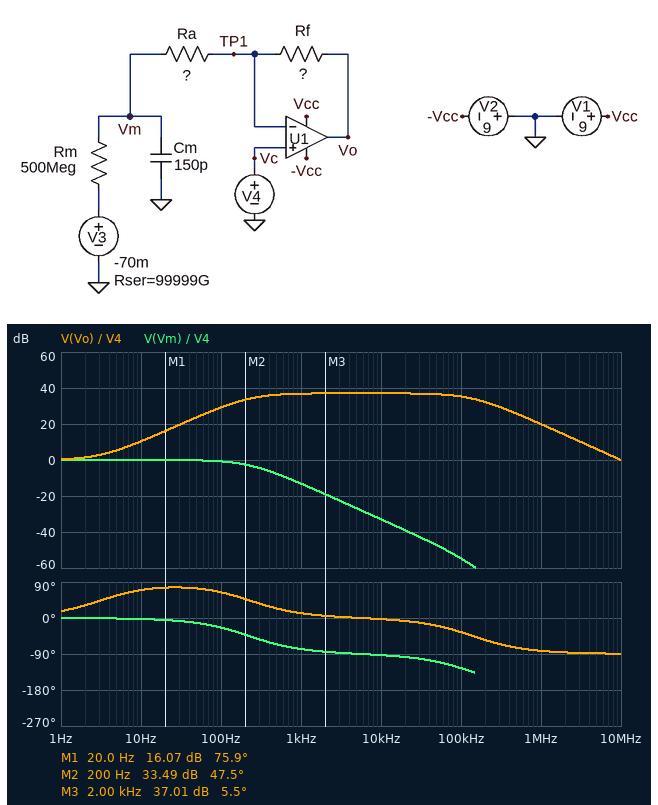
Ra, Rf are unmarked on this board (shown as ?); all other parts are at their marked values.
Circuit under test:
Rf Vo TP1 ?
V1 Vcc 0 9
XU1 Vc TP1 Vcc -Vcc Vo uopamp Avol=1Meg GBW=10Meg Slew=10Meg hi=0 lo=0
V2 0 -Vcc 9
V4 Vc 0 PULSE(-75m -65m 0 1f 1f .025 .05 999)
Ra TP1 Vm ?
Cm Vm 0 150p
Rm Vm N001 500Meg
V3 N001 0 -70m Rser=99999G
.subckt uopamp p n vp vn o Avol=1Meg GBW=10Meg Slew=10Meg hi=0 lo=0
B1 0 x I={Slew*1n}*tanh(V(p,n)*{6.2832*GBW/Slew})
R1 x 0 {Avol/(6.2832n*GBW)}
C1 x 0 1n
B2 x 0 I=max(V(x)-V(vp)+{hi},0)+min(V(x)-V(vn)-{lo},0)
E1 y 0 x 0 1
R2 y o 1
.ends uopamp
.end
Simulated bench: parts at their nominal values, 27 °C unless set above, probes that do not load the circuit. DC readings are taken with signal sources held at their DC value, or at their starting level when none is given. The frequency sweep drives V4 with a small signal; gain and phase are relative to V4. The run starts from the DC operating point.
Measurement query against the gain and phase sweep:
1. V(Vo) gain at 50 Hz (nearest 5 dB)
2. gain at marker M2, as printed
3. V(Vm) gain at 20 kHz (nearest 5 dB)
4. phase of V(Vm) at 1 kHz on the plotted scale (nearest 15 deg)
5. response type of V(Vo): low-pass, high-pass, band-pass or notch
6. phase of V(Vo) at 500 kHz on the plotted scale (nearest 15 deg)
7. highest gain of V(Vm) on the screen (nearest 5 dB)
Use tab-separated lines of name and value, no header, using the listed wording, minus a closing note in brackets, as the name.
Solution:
V(Vo) gain at 50 Hz	25 dB
gain at marker M2, as printed	33.49 dB
V(Vm) gain at 20 kHz	-40 dB
phase of V(Vm) at 1 kHz on the plotted scale	-75 deg
response type of V(Vo): low-pass, high-pass, band-pass or notch	band-pass
phase of V(Vo) at 500 kHz on the plotted scale	-75 deg
highest gain of V(Vm) on the screen	0 dB
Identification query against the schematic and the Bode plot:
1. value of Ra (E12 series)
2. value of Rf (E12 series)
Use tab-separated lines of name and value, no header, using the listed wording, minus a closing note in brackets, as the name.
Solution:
value of Ra	4.7 MΩ
value of Rf	330 MΩ
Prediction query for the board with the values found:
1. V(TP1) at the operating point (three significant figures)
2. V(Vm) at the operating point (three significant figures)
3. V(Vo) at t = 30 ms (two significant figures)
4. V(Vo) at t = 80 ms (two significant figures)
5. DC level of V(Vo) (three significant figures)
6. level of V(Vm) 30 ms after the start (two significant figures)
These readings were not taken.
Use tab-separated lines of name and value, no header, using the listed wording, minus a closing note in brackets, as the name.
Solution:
V(TP1) at the operating point	-75.0 mV
V(Vm) at the operating point	-75.0 mV
V(Vo) at t = 30 ms	-76 mV
V(Vo) at t = 80 ms	-76 mV
DC level of V(Vo)	-75.0 mV
level of V(Vm) 30 ms after the start	-75 mV
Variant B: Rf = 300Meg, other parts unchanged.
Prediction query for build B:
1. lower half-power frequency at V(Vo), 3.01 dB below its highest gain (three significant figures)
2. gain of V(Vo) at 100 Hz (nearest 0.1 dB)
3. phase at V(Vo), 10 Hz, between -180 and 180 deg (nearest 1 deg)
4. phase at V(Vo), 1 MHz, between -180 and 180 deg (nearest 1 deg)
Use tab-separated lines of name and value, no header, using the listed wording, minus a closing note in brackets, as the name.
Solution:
lower half-power frequency at V(Vo), 3.01 dB below its highest gain	225 Hz
gain of V(Vo) at 100 Hz	28.4 dB
phase at V(Vo), 10 Hz, between -180 and 180 deg	68 deg
phase at V(Vo), 1 MHz, between -180 and 180 deg	-81 deg
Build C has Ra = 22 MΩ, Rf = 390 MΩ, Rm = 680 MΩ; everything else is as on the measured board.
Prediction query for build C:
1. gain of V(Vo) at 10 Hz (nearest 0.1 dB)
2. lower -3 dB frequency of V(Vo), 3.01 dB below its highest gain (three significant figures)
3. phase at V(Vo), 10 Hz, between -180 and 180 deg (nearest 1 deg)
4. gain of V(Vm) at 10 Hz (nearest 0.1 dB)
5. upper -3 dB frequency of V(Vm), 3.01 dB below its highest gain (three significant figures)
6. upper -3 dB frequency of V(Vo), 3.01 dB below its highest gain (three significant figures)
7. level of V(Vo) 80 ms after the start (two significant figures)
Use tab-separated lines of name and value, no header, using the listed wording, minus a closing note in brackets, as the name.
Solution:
gain of V(Vo) at 10 Hz	11.9 dB
lower -3 dB frequency of V(Vo), 3.01 dB below its highest gain	48.1 Hz
phase at V(Vo), 10 Hz, between -180 and 180 deg	64 deg
gain of V(Vm) at 10 Hz	-0.2 dB
upper -3 dB frequency of V(Vm), 3.01 dB below its highest gain	48.2 Hz
upper -3 dB frequency of V(Vo), 3.01 dB below its highest gain	534 kHz
level of V(Vo) 80 ms after the start	-110 mV
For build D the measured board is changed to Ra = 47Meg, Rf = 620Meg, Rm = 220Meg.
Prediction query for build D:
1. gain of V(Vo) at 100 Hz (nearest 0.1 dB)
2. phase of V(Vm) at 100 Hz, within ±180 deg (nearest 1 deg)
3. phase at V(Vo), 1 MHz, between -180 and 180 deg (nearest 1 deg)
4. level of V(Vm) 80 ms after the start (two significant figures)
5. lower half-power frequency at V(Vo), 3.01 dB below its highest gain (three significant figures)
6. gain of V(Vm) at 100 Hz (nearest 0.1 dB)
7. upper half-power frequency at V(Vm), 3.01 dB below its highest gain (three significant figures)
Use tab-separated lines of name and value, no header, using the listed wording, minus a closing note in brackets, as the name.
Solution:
gain of V(Vo) at 100 Hz	22.8 dB
phase of V(Vm) at 100 Hz, within ±180 deg	-77 deg
phase at V(Vo), 1 MHz, between -180 and 180 deg	-55 deg
level of V(Vm) 80 ms after the start	-70 mV
lower half-power frequency at V(Vo), 3.01 dB below its highest gain	22.5 Hz
gain of V(Vm) at 100 Hz	-13.1 dB
upper half-power frequency at V(Vm), 3.01 dB below its highest gain	22.6 Hz
